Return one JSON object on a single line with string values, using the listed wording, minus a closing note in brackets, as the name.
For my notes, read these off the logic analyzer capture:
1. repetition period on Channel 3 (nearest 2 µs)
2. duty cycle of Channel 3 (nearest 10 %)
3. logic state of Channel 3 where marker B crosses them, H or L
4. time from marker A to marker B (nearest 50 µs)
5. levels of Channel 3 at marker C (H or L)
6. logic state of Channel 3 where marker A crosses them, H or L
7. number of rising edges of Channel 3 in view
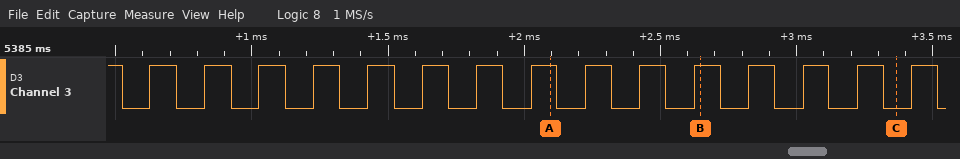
{"repetition period on Channel 3": "200 µs", "duty cycle of Channel 3": "50 %", "logic state of Channel 3 where marker B crosses them, H or L": "Channel 3=H", "time from marker A to marker B": "550 µs", "levels of Channel 3 at marker C": "Channel 3=L", "logic state of Channel 3 where marker A crosses them, H or L": "Channel 3=H", "number of rising edges of Channel 3 in view": "15"}
